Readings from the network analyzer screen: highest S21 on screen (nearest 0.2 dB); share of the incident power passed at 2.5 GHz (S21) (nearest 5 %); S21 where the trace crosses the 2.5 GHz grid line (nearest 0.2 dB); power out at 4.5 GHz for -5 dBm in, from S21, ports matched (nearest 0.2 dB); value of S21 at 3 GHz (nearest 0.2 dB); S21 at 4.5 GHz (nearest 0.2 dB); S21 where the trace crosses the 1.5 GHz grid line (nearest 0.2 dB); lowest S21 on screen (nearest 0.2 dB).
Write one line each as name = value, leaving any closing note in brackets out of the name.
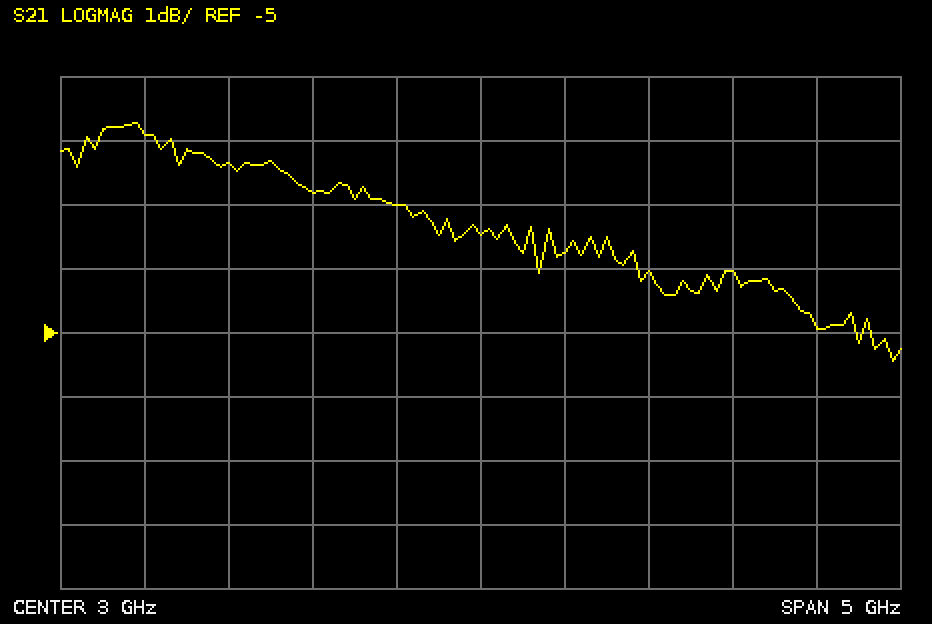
highest S21 on screen = -1.8 dB
share of the incident power passed at 2.5 GHz (S21) = 50 %
S21 where the trace crosses the 2.5 GHz grid line = -3.0 dB
power out at 4.5 GHz for -5 dBm in, from S21, ports matched = -9.0 dBm
value of S21 at 3 GHz = -3.4 dB
S21 at 4.5 GHz = -4.0 dB
S21 where the trace crosses the 1.5 GHz grid line = -2.4 dB
lowest S21 on screen = -5.4 dB
